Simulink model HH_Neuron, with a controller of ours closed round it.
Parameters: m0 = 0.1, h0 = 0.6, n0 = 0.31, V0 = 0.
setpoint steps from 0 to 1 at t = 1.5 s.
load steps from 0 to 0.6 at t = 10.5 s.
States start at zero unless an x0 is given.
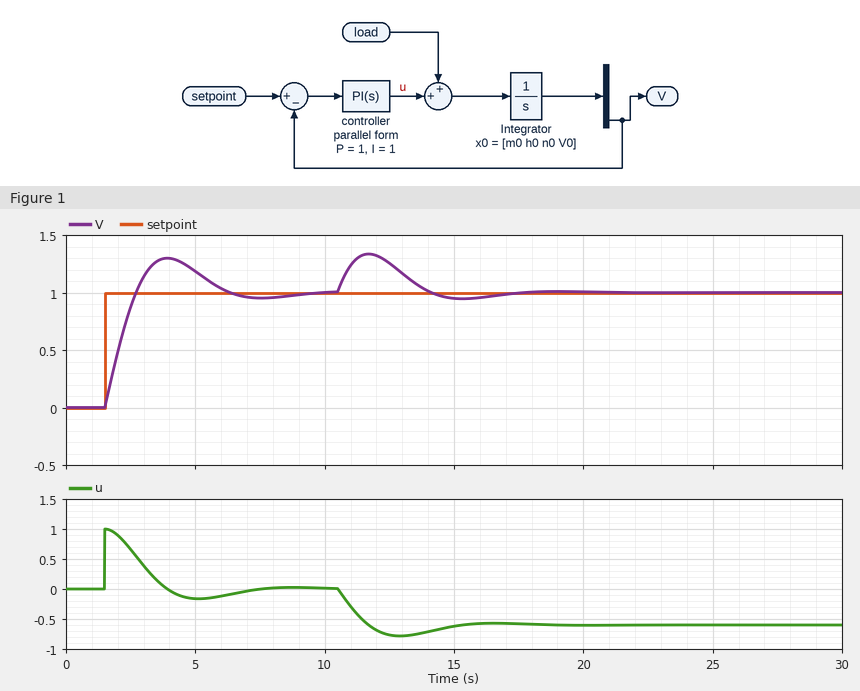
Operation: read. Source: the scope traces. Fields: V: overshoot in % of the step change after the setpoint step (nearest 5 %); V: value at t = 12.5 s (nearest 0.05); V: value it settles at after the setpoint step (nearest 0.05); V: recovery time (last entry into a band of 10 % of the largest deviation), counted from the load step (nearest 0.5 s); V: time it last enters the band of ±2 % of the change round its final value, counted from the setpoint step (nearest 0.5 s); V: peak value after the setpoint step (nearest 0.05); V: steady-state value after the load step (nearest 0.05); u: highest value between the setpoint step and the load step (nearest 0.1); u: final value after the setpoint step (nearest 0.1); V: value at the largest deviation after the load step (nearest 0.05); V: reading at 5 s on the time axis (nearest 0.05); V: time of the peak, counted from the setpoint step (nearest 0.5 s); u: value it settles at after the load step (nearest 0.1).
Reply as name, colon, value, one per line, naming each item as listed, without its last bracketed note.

V: overshoot in % of the step change after the setpoint step: 30 %
V: value at t = 12.5 s: 1.25
V: value it settles at after the setpoint step: 1.00
V: recovery time (last entry into a band of 10 % of the largest deviation), counted from the load step: 6.0 s
V: time it last enters the band of ±2 % of the change round its final value, counted from the setpoint step: 7.5 s
V: peak value after the setpoint step: 1.30
V: steady-state value after the load step: 1.00
u: highest value between the setpoint step and the load step: 1.0
u: final value after the setpoint step: 0.0
V: value at the largest deviation after the load step: 1.35
V: reading at 5 s on the time axis: 1.20
V: time of the peak, counted from the setpoint step: 2.5 s
u: value it settles at after the load step: -0.6
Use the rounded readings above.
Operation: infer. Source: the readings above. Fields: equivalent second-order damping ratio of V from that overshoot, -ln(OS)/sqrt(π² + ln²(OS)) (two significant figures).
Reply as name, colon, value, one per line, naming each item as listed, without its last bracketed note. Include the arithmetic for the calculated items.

equivalent second-order damping ratio of V from that overshoot, -ln(OS)/sqrt(π² + ln²(OS)): ln(0.3) = -1.204; 1.204 / sqrt(9.870 + 1.450) = 0.36
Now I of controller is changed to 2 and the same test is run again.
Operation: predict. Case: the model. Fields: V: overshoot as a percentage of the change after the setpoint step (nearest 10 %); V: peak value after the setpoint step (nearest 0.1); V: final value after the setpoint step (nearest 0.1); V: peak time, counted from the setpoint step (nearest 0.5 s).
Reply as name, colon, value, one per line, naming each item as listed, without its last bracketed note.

V: overshoot as a percentage of the change after the setpoint step: 40 %
V: peak value after the setpoint step: 1.4
V: final value after the setpoint step: 1.0
V: peak time, counted from the setpoint step: 2.0 s
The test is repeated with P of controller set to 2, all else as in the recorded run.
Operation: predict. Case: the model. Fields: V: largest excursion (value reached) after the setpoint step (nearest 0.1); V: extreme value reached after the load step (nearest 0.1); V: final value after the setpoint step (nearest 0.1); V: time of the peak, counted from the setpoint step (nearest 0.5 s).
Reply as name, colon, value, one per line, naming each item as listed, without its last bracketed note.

V: largest excursion (value reached) after the setpoint step: 1.1
V: extreme value reached after the load step: 1.2
V: final value after the setpoint step: 1.0
V: time of the peak, counted from the setpoint step: 2.0 s
